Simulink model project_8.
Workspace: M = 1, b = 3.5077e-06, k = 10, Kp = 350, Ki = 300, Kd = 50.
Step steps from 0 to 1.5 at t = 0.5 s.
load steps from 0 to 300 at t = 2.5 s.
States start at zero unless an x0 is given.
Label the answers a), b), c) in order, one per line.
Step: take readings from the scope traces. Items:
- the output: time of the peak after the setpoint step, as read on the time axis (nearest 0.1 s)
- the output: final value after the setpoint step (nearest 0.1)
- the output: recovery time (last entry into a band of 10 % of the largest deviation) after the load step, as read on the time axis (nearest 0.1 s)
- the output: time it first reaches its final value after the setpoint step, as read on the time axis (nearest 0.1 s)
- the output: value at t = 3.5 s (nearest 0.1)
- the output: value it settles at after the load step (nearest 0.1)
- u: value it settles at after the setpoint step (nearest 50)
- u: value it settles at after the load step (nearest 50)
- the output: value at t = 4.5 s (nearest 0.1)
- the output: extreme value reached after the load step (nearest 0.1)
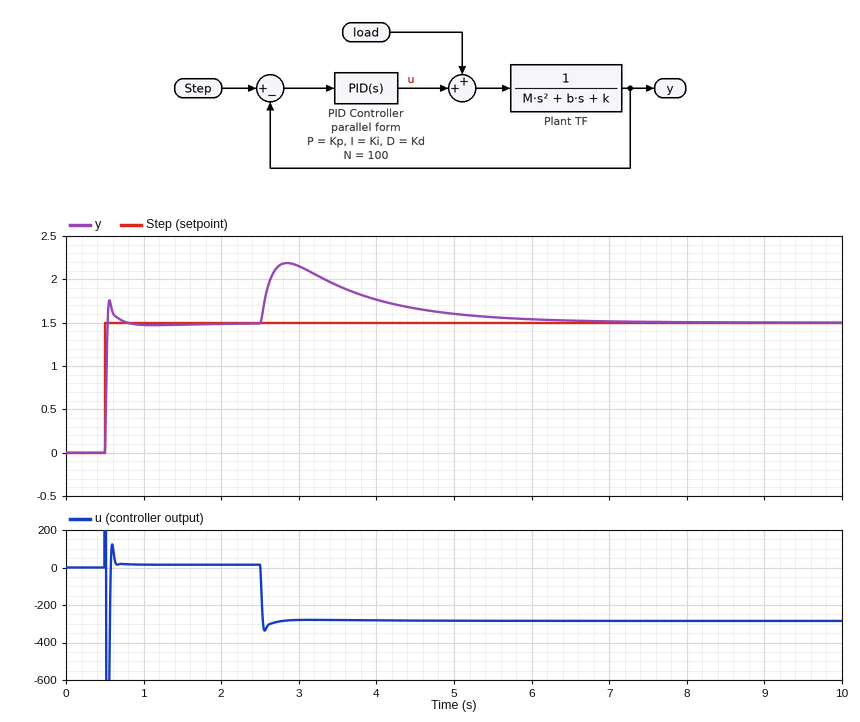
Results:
a) 0.6 s
b) 1.5
c) 5.4 s
d) 0.5 s
e) 1.9
f) 1.5
g) 0
h) -300
i) 1.7
j) 2.2
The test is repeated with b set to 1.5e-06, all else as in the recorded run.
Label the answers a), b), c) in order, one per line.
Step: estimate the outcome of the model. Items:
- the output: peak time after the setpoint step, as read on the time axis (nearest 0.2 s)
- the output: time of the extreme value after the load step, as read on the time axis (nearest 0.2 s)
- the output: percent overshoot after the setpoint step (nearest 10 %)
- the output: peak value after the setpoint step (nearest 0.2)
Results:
a) 0.6 s
b) 2.8 s
c) 20 %
d) 1.8
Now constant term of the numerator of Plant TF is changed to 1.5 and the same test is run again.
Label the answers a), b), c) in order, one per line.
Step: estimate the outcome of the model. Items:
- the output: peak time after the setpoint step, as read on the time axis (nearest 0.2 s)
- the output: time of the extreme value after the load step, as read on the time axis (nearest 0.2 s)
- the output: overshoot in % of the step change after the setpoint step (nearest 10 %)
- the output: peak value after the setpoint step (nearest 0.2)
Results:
a) 0.6 s
b) 2.8 s
c) 20 %
d) 1.8
